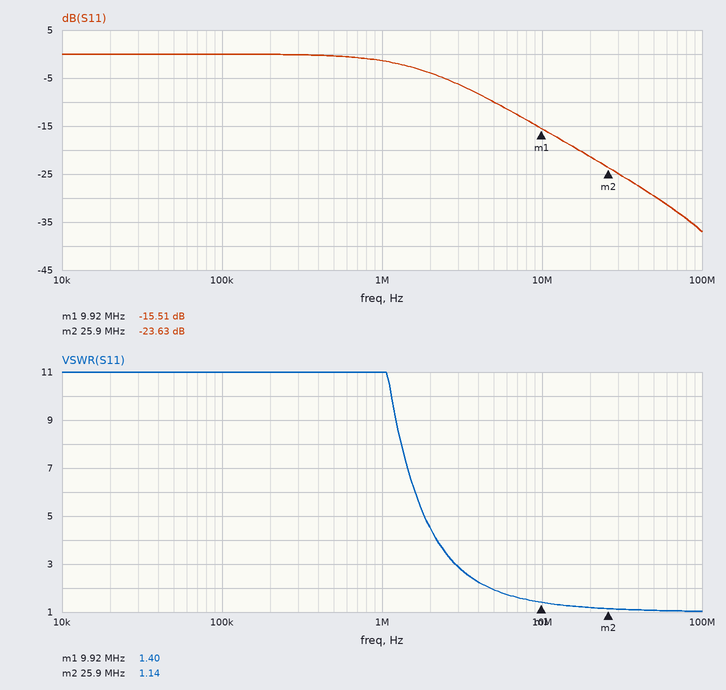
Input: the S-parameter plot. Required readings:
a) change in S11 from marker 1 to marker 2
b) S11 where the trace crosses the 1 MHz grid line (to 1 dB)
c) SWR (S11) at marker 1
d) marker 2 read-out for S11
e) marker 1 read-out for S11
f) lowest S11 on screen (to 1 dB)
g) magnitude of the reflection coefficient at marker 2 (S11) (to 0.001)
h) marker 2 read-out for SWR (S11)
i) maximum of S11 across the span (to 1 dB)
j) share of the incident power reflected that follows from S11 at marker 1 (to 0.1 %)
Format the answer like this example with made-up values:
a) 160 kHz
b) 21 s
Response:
a) -8.12 dB
b) -1 dB
c) 1.40
d) -23.63 dB
e) -15.51 dB
f) -37 dB
g) 0.066
h) 1.14
i) 0 dB
j) 2.8 %
